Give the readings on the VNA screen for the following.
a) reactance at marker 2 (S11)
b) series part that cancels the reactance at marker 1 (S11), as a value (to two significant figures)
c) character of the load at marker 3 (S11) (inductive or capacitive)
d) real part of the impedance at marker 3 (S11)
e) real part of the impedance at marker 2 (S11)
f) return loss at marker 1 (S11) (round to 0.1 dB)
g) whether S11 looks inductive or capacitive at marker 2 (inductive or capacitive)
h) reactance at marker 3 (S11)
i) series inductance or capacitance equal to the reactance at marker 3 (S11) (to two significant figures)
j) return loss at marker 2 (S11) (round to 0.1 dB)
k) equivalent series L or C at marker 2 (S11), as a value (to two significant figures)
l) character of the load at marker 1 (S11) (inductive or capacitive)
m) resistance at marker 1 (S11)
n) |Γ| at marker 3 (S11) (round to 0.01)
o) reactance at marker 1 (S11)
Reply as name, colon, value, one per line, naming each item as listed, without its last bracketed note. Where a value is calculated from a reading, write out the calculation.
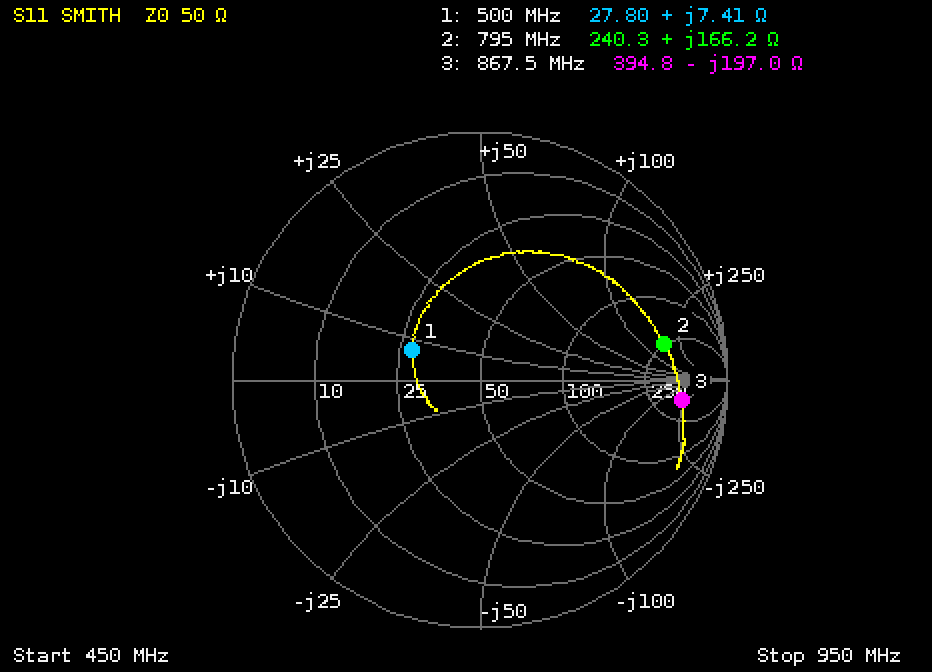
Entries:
reactance at marker 2: +166.2 Ω
series part that cancels the reactance at marker 1 (S11), as a value: C = 1/(2π × 500 MHz × 7.41 Ω) ≈ 43 pF
character of the load at marker 3 (S11): capacitive
real part of the impedance at marker 3: 394.8 Ω
real part of the impedance at marker 2: 240.3 Ω
return loss at marker 1 (S11): 10.5 dB
whether S11 looks inductive or capacitive at marker 2: inductive
reactance at marker 3: -197.0 Ω
series inductance or capacitance equal to the reactance at marker 3 (S11): C = 1/(2π × 867.5 MHz × 197 Ω) ≈ 931 fF, so 930 fF to two significant figures
return loss at marker 2 (S11): 2.4 dB
equivalent series L or C at marker 2 (S11), as a value: L = 166.2 Ω/(2π × 795 MHz) ≈ 33 nH
character of the load at marker 1 (S11): inductive
resistance at marker 1: 27.80 Ω
|Γ| at marker 3 (S11): 0.82
reactance at marker 1: +7.41 Ω
